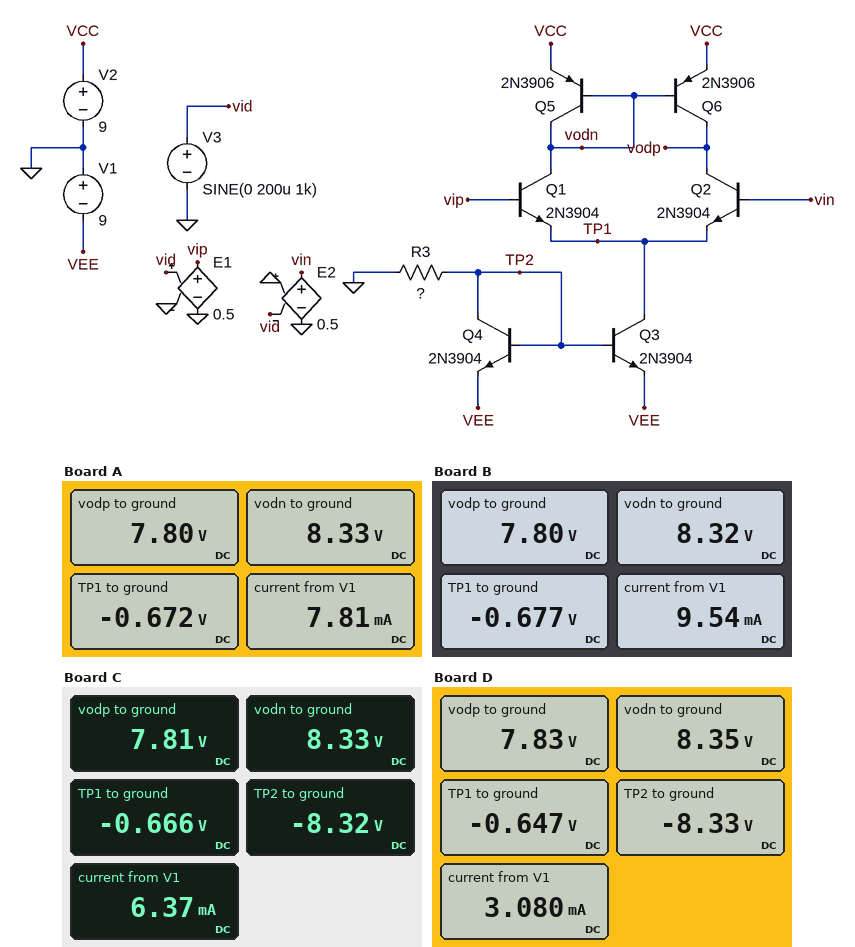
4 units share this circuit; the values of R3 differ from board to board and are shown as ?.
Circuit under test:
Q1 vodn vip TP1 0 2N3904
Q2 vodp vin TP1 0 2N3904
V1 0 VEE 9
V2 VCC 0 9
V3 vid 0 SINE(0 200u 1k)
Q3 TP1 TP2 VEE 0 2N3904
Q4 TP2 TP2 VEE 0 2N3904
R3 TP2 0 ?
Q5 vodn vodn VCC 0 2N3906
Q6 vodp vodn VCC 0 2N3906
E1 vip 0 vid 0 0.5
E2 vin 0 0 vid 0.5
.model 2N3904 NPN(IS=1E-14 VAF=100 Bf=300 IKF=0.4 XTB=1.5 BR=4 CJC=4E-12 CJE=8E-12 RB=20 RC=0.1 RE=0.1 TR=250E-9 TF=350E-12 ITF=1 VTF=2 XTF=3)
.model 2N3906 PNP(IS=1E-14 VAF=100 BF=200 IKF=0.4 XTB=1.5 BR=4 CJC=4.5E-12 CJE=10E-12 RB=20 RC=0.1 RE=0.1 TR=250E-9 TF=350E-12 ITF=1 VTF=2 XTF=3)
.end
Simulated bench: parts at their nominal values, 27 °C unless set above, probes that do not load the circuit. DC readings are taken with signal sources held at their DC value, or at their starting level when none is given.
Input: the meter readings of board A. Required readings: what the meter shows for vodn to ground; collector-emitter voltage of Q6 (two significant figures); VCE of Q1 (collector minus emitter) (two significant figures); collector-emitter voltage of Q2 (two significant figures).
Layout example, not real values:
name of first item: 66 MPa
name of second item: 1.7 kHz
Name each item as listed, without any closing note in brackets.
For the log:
what the meter shows for vodn to ground: 8.33 V
collector-emitter voltage of Q6: -1.2 V
VCE of Q1 (collector minus emitter): 9.0 V
collector-emitter voltage of Q2: 8.5 V
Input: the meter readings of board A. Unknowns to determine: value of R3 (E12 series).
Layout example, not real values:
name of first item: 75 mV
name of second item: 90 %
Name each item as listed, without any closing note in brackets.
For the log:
value of R3: 2.2 kΩ
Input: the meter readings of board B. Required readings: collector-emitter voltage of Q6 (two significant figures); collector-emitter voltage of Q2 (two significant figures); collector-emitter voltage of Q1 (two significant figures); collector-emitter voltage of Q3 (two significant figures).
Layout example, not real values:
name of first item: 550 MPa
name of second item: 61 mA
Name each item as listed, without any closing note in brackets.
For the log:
collector-emitter voltage of Q6: -1.2 V
collector-emitter voltage of Q2: 8.5 V
collector-emitter voltage of Q1: 9.0 V
collector-emitter voltage of Q3: 8.3 V
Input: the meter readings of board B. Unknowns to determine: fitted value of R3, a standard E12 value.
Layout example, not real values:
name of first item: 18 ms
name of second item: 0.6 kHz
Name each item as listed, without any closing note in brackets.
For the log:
fitted value of R3, a standard E12 value: 1.8 kΩ
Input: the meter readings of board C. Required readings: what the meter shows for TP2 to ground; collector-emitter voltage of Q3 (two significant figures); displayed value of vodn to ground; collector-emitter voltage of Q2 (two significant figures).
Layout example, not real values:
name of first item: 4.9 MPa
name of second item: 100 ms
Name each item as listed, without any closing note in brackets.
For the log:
what the meter shows for TP2 to ground: -8.32 V
collector-emitter voltage of Q3: 8.3 V
displayed value of vodn to ground: 8.33 V
collector-emitter voltage of Q2: 8.5 V
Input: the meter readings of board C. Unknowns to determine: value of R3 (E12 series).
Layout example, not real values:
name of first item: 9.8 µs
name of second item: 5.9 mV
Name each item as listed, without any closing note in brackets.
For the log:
value of R3: 2.7 kΩ
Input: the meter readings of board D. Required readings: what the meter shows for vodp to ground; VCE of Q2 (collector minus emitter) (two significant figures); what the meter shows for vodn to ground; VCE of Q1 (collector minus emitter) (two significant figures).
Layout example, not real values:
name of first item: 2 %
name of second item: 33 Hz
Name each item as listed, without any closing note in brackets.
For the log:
what the meter shows for vodp to ground: 7.83 V
VCE of Q2 (collector minus emitter): 8.5 V
what the meter shows for vodn to ground: 8.35 V
VCE of Q1 (collector minus emitter): 9.0 V
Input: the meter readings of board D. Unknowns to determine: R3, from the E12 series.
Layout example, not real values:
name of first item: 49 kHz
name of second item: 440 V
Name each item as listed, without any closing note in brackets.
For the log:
R3, from the E12 series: 5.6 kΩ
